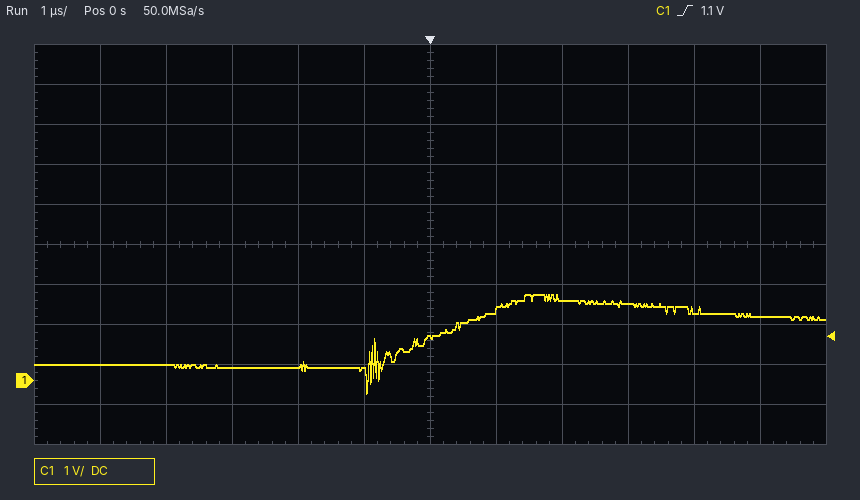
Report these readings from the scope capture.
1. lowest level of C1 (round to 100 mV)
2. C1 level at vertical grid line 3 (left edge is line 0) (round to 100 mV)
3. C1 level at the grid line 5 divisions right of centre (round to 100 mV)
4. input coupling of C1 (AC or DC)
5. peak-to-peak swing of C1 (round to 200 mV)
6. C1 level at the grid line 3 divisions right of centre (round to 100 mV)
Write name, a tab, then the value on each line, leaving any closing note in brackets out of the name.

lowest level of C1	-300 mV
C1 level at vertical grid line 3 (left edge is line 0)	300 mV
C1 level at the grid line 5 divisions right of centre	1.6 V
input coupling of C1	DC
peak-to-peak swing of C1	2.4 V
C1 level at the grid line 3 divisions right of centre	1.9 V
